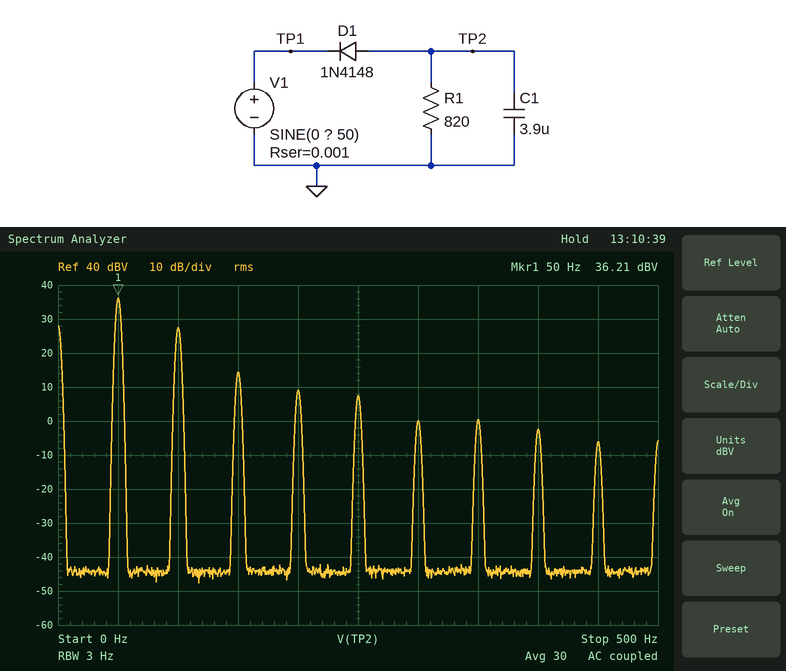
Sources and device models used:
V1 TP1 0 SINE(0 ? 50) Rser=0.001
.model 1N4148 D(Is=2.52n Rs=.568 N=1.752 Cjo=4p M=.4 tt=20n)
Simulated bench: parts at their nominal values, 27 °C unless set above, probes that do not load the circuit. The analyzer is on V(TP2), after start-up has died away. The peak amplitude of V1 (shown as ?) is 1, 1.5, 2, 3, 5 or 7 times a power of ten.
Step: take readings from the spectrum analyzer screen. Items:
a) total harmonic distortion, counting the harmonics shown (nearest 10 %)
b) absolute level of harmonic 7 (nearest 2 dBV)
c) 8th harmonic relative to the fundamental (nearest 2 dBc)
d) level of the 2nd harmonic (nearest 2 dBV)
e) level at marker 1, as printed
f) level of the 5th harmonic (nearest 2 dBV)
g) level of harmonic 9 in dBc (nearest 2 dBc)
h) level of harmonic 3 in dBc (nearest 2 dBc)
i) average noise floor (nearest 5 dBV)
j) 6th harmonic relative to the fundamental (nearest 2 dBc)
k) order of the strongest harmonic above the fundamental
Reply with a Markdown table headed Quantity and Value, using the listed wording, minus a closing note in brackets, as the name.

| Quantity | Value |
|---|---|
| total harmonic distortion, counting the harmonics shown | 40 % |
| absolute level of harmonic 7 | 0 dBV |
| 8th harmonic relative to the fundamental | -38 dBc |
| level of the 2nd harmonic | 28 dBV |
| level at marker 1, as printed | 36.21 dBV |
| level of the 5th harmonic | 8 dBV |
| level of harmonic 9 in dBc | -42 dBc |
| level of harmonic 3 in dBc | -22 dBc |
| average noise floor | -45 dBV |
| 6th harmonic relative to the fundamental | -36 dBc |
| order of the strongest harmonic above the fundamental | 2 |
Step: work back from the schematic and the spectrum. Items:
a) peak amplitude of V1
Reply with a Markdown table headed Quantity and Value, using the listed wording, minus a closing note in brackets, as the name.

| Quantity | Value |
|---|---|
| peak amplitude of V1 | 200 V |
